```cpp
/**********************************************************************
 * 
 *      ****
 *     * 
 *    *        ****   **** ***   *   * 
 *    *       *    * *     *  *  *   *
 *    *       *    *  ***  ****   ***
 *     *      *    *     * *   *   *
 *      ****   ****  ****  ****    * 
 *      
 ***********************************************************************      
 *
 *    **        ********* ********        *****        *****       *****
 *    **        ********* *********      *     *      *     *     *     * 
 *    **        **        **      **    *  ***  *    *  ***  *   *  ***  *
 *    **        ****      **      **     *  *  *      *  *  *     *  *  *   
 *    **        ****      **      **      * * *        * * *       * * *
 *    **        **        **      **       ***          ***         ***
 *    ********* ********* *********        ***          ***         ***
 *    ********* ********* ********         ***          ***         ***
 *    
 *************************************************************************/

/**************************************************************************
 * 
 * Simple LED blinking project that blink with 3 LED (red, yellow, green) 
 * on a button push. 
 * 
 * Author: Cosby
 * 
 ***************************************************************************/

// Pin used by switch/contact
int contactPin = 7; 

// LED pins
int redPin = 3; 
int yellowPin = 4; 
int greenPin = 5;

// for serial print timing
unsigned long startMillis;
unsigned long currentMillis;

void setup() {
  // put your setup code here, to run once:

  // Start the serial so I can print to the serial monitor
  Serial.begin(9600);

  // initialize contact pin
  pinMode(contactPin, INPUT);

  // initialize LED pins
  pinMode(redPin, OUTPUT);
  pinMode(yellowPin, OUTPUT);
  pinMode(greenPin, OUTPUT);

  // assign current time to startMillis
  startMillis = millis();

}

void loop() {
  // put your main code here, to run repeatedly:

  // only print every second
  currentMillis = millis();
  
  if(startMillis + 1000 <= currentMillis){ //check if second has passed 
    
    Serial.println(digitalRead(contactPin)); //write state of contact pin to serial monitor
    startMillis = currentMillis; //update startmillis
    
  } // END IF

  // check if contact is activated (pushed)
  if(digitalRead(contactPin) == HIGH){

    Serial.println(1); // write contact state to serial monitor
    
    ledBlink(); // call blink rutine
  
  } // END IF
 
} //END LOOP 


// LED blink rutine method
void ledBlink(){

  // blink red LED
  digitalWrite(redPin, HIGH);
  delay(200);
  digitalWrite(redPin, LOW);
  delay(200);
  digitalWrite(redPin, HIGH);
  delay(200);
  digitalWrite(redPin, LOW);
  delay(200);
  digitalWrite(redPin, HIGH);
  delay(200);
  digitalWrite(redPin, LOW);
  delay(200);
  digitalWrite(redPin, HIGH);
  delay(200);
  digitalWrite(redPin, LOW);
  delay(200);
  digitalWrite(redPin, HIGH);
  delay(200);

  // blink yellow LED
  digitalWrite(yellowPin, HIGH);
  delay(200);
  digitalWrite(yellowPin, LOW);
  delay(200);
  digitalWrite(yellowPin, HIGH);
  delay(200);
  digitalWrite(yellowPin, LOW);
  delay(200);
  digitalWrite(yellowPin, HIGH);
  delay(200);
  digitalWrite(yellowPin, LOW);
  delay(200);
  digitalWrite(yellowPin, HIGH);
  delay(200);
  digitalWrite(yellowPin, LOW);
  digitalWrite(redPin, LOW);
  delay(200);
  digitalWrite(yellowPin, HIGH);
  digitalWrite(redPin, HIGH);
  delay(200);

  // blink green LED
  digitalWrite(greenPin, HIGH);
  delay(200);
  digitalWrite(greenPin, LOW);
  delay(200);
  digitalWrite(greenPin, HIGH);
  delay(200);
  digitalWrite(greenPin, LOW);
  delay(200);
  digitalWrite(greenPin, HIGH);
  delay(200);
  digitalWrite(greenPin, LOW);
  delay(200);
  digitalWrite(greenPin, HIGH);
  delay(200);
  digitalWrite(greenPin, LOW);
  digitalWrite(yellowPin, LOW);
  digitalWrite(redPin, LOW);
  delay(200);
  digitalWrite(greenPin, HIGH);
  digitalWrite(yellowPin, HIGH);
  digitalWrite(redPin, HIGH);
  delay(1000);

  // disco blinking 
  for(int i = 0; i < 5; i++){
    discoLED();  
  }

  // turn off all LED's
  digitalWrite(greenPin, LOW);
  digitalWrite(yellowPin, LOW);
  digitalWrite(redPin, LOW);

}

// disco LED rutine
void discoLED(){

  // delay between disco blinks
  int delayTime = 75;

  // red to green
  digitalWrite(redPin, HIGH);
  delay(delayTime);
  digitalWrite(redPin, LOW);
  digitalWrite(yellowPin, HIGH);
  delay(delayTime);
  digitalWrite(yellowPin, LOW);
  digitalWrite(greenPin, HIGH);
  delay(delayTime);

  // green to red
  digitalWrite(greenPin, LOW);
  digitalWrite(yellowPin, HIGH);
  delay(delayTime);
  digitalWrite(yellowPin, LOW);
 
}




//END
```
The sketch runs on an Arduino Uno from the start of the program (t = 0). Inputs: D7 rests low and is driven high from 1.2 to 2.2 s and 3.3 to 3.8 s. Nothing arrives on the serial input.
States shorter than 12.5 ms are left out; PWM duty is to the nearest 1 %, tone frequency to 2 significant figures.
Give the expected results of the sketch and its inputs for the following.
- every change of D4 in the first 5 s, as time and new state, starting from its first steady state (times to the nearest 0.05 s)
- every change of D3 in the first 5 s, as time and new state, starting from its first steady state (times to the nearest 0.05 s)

0 s low; 3 s high; 3.2 s low; 3.4 s high; 3.6 s low; 3.8 s high; 4 s low; 4.2 s high; 4.4 s low; 4.6 s high
0 s low; 1.2 s high; 1.4 s low; 1.6 s high; 1.8 s low; 2 s high; 2.2 s low; 2.4 s high; 2.6 s low; 2.8 s high; 4.4 s low; 4.6 s high
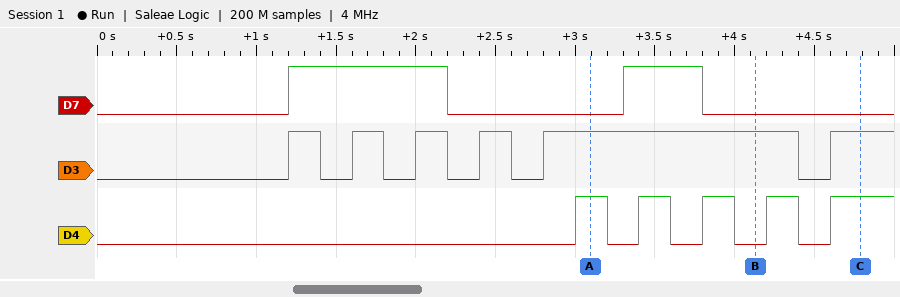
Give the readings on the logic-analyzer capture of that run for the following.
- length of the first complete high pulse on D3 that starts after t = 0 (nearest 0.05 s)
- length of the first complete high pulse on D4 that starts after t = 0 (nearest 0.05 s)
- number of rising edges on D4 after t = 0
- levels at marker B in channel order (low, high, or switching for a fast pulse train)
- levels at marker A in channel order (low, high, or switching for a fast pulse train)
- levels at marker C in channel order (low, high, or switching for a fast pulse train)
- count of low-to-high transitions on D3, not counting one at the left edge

0.20 s
0.20 s
5
D7 low, D3 high, D4 low
D7 low, D3 high, D4 high
D7 low, D3 high, D4 high
6
